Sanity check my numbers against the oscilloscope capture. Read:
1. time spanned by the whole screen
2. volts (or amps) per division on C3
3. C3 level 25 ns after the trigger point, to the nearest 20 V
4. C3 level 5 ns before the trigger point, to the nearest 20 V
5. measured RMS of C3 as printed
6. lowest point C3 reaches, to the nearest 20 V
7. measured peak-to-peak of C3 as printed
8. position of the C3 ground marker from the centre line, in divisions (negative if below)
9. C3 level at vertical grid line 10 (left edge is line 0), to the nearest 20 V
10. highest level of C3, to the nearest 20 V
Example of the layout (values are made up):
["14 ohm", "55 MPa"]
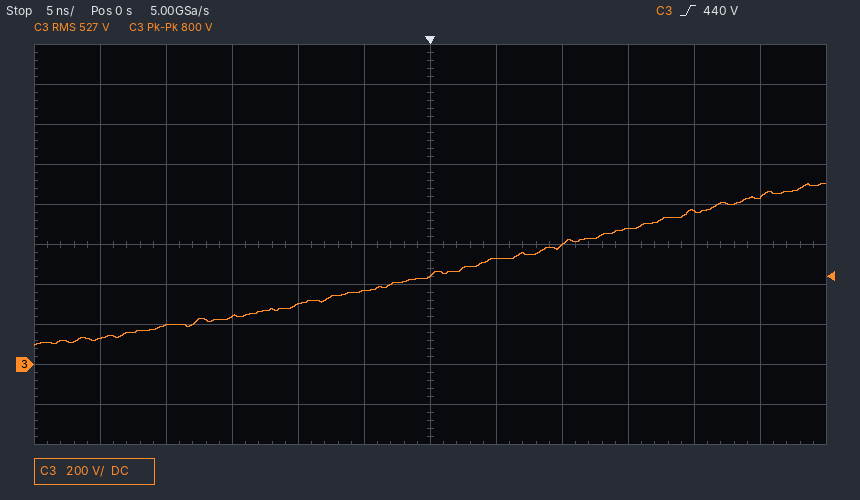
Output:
["60 ns", "200 V", "840 V", "360 V", "527 V", "100 V", "800 V", "-3.0 div", "760 V", "900 V"]
